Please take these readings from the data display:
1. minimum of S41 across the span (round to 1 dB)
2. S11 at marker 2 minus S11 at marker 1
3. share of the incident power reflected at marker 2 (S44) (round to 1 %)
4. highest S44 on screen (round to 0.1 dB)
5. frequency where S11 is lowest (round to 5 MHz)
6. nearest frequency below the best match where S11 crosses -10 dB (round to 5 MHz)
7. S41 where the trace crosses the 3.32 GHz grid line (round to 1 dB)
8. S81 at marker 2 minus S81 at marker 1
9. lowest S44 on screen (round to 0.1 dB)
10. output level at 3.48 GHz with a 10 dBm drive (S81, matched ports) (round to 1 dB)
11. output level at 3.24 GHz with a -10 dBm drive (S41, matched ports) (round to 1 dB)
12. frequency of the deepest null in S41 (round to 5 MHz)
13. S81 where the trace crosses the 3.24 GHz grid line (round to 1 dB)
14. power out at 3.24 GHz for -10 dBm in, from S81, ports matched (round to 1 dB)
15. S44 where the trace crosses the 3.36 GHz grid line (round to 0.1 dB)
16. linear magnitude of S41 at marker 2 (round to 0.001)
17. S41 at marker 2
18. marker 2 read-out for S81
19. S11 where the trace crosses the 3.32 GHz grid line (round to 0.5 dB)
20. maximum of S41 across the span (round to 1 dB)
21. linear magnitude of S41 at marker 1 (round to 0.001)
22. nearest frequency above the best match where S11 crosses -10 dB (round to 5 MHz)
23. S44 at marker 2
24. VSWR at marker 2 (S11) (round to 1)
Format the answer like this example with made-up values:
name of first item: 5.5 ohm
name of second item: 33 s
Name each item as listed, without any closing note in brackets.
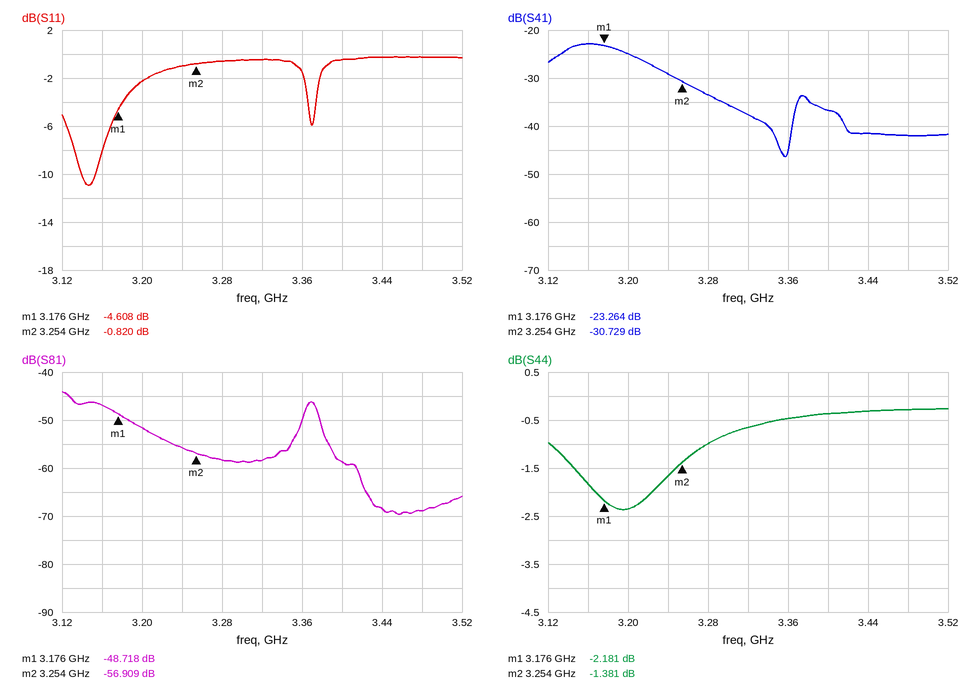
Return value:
minimum of S41 across the span: -46 dB
S11 at marker 2 minus S11 at marker 1: 3.788 dB
share of the incident power reflected at marker 2 (S44): 73 %
highest S44 on screen: -0.3 dB
frequency where S11 is lowest: 3.145 GHz
nearest frequency below the best match where S11 crosses -10 dB: 3.140 GHz
S41 where the trace crosses the 3.32 GHz grid line: -38 dB
S81 at marker 2 minus S81 at marker 1: -8.191 dB
lowest S44 on screen: -2.4 dB
output level at 3.48 GHz with a 10 dBm drive (S81, matched ports): -59 dBm
output level at 3.24 GHz with a -10 dBm drive (S41, matched ports): -39 dBm
frequency of the deepest null in S41: 3.355 GHz
S81 where the trace crosses the 3.24 GHz grid line: -56 dB
power out at 3.24 GHz for -10 dBm in, from S81, ports matched: -66 dBm
S44 where the trace crosses the 3.36 GHz grid line: -0.5 dB
linear magnitude of S41 at marker 2: 0.029
S41 at marker 2: -30.729 dB
marker 2 read-out for S81: -56.909 dB
S11 where the trace crosses the 3.32 GHz grid line: -0.5 dB
maximum of S41 across the span: -23 dB
linear magnitude of S41 at marker 1: 0.069
nearest frequency above the best match where S11 crosses -10 dB: 3.155 GHz
S44 at marker 2: -1.381 dB
VSWR at marker 2 (S11): 21
